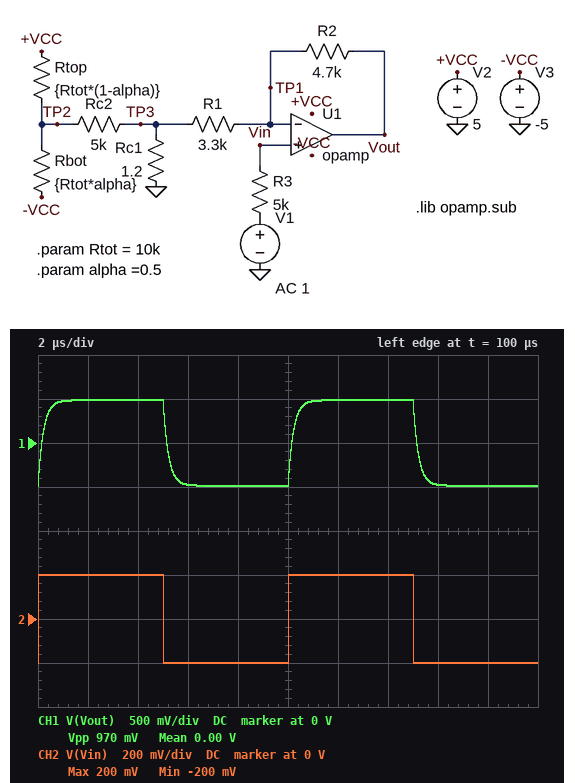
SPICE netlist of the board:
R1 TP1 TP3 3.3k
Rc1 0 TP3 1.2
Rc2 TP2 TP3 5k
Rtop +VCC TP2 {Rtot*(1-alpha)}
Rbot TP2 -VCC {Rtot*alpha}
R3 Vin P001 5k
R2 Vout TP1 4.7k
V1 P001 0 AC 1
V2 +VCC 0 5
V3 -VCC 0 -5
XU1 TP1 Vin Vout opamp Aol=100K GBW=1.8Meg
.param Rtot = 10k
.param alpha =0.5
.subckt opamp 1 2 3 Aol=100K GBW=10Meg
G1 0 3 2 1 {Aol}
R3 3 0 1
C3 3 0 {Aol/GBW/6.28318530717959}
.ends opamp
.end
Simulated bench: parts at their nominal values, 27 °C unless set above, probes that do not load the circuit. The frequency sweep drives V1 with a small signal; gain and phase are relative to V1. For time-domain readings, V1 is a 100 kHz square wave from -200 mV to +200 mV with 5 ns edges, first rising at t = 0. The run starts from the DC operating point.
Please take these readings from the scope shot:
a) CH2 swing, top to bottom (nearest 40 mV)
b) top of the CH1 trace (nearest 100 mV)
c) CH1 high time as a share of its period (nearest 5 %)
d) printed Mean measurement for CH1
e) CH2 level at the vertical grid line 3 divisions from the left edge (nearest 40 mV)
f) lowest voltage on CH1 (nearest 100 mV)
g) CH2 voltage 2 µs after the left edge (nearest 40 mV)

400 mV
500 mV
50 %
0.00 V
-200 mV
-500 mV
200 mV
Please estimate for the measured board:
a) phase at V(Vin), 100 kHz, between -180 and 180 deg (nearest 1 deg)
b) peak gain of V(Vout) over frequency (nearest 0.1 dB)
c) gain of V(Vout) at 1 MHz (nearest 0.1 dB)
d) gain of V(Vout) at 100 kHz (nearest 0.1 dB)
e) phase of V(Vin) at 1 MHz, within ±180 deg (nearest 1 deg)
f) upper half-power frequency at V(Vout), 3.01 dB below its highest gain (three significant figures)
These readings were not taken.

0 deg
7.7 dB
3.2 dB
7.6 dB
0 deg
743 kHz
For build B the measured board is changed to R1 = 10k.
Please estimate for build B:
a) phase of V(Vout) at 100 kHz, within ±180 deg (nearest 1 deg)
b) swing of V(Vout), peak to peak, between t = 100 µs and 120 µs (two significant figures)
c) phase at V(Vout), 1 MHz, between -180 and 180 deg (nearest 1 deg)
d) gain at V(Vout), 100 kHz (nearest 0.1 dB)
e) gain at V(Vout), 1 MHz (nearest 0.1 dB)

-5 deg
590 mV
-39 deg
3.3 dB
1.1 dB
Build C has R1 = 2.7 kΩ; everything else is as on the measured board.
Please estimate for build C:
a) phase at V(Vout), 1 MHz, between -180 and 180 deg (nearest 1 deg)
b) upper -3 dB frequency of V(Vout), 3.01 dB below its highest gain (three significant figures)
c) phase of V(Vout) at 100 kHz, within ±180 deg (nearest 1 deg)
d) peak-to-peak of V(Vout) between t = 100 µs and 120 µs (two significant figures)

-57 deg
657 kHz
-9 deg
1.1 V
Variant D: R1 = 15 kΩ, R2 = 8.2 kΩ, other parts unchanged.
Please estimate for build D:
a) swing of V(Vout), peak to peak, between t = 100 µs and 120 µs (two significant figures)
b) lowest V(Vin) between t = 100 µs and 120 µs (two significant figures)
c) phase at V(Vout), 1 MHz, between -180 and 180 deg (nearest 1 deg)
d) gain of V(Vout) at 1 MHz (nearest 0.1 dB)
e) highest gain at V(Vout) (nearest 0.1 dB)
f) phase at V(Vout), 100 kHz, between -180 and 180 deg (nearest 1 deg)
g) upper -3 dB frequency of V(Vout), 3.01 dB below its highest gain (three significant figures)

620 mV
-200 mV
-41 deg
1.4 dB
3.8 dB
-5 deg
1.16 MHz
